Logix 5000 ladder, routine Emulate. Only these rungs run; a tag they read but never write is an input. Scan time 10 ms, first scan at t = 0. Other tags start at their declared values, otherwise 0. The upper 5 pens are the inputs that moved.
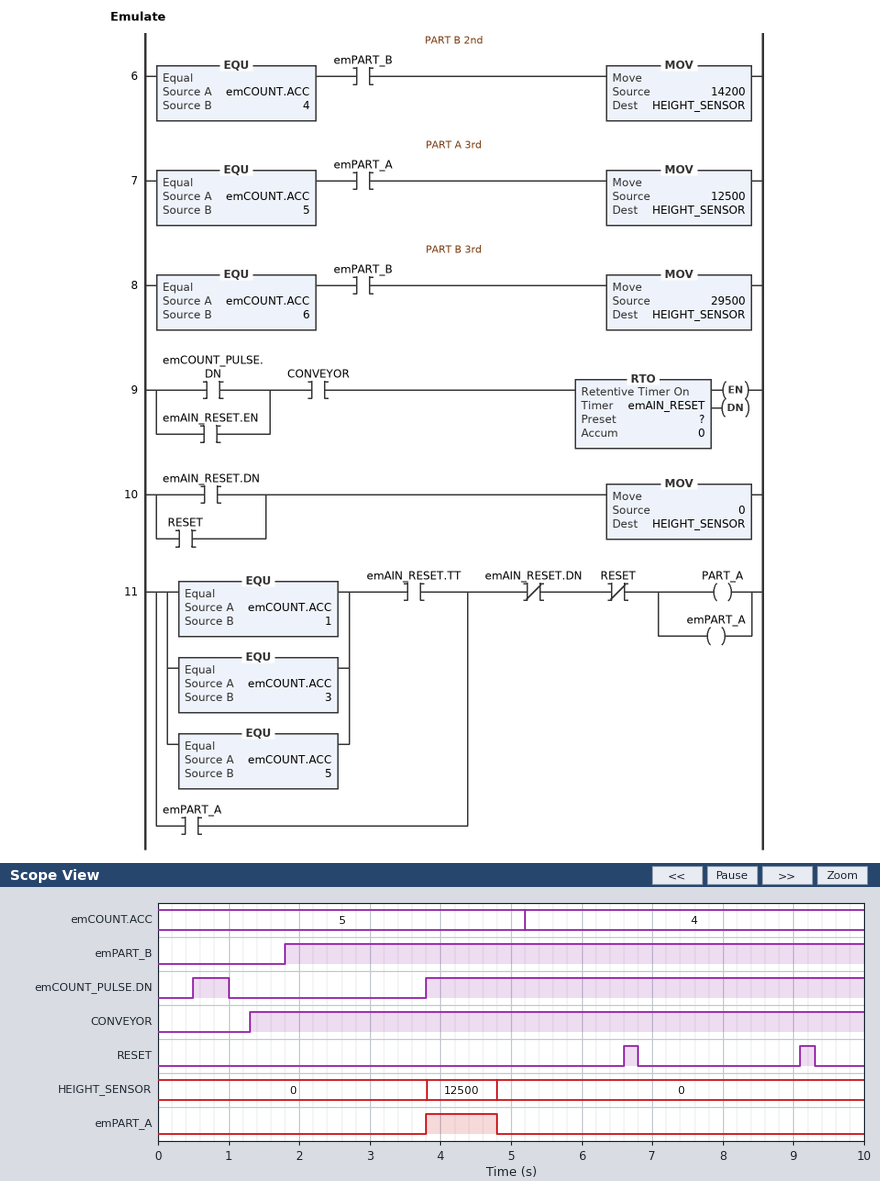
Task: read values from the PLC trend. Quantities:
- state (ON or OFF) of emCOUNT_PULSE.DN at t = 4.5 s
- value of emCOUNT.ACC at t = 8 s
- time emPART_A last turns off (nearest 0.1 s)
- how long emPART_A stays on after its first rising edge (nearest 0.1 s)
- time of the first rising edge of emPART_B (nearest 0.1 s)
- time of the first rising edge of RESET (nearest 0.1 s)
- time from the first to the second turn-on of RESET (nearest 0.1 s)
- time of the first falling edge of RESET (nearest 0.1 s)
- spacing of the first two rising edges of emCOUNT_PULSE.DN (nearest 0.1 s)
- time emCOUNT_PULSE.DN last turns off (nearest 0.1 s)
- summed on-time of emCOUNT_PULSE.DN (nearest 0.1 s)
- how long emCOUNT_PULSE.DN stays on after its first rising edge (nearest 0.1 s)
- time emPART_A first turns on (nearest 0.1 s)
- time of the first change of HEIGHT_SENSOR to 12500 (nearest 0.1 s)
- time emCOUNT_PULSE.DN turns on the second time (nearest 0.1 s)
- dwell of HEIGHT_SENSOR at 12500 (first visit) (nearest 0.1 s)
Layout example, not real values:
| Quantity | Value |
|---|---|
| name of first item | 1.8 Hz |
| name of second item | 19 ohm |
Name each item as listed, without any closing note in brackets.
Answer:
| Quantity | Value |
|---|---|
| state (ON or OFF) of emCOUNT_PULSE.DN at t = 4.5 s | ON |
| value of emCOUNT.ACC at t = 8 s | 4 |
| time emPART_A last turns off | 4.8 s |
| how long emPART_A stays on after its first rising edge | 1.0 s |
| time of the first rising edge of emPART_B | 1.8 s |
| time of the first rising edge of RESET | 6.6 s |
| time from the first to the second turn-on of RESET | 2.5 s |
| time of the first falling edge of RESET | 6.8 s |
| spacing of the first two rising edges of emCOUNT_PULSE.DN | 3.3 s |
| time emCOUNT_PULSE.DN last turns off | 1.0 s |
| summed on-time of emCOUNT_PULSE.DN | 6.7 s |
| how long emCOUNT_PULSE.DN stays on after its first rising edge | 0.5 s |
| time emPART_A first turns on | 3.8 s |
| time of the first change of HEIGHT_SENSOR to 12500 | 3.8 s |
| time emCOUNT_PULSE.DN turns on the second time | 3.8 s |
| dwell of HEIGHT_SENSOR at 12500 (first visit) | 1.0 s |
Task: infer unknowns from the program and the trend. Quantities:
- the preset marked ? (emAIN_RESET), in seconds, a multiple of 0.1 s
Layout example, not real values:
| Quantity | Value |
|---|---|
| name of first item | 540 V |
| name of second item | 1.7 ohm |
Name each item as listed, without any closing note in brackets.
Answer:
| Quantity | Value |
|---|---|
| the preset marked ? (emAIN_RESET), in seconds, a multiple of 0.1 s | 1.0 s |
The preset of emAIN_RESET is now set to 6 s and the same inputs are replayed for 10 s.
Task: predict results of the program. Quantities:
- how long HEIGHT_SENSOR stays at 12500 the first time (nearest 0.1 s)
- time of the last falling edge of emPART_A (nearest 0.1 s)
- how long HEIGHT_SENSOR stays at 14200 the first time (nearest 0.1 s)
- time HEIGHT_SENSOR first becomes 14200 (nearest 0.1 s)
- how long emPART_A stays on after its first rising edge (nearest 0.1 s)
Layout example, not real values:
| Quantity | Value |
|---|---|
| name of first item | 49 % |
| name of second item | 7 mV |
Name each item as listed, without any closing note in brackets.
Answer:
| Quantity | Value |
|---|---|
| how long HEIGHT_SENSOR stays at 12500 the first time | 1.4 s |
| time of the last falling edge of emPART_A | 6.6 s |
| how long HEIGHT_SENSOR stays at 14200 the first time | 1.4 s |
| time HEIGHT_SENSOR first becomes 14200 | 5.2 s |
| how long emPART_A stays on after its first rising edge | 2.8 s |
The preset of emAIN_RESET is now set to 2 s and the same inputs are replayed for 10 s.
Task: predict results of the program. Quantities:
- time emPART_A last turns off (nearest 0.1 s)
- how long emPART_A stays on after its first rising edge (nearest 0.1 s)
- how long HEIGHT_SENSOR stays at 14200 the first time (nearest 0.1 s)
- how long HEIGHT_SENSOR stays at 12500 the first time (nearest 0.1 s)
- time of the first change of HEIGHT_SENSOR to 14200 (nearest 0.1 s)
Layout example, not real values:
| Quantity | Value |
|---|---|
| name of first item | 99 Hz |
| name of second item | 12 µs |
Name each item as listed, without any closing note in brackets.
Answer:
| Quantity | Value |
|---|---|
| time emPART_A last turns off | 5.8 s |
| how long emPART_A stays on after its first rising edge | 2.0 s |
| how long HEIGHT_SENSOR stays at 14200 the first time | 0.6 s |
| how long HEIGHT_SENSOR stays at 12500 the first time | 1.4 s |
| time of the first change of HEIGHT_SENSOR to 14200 | 5.2 s |
